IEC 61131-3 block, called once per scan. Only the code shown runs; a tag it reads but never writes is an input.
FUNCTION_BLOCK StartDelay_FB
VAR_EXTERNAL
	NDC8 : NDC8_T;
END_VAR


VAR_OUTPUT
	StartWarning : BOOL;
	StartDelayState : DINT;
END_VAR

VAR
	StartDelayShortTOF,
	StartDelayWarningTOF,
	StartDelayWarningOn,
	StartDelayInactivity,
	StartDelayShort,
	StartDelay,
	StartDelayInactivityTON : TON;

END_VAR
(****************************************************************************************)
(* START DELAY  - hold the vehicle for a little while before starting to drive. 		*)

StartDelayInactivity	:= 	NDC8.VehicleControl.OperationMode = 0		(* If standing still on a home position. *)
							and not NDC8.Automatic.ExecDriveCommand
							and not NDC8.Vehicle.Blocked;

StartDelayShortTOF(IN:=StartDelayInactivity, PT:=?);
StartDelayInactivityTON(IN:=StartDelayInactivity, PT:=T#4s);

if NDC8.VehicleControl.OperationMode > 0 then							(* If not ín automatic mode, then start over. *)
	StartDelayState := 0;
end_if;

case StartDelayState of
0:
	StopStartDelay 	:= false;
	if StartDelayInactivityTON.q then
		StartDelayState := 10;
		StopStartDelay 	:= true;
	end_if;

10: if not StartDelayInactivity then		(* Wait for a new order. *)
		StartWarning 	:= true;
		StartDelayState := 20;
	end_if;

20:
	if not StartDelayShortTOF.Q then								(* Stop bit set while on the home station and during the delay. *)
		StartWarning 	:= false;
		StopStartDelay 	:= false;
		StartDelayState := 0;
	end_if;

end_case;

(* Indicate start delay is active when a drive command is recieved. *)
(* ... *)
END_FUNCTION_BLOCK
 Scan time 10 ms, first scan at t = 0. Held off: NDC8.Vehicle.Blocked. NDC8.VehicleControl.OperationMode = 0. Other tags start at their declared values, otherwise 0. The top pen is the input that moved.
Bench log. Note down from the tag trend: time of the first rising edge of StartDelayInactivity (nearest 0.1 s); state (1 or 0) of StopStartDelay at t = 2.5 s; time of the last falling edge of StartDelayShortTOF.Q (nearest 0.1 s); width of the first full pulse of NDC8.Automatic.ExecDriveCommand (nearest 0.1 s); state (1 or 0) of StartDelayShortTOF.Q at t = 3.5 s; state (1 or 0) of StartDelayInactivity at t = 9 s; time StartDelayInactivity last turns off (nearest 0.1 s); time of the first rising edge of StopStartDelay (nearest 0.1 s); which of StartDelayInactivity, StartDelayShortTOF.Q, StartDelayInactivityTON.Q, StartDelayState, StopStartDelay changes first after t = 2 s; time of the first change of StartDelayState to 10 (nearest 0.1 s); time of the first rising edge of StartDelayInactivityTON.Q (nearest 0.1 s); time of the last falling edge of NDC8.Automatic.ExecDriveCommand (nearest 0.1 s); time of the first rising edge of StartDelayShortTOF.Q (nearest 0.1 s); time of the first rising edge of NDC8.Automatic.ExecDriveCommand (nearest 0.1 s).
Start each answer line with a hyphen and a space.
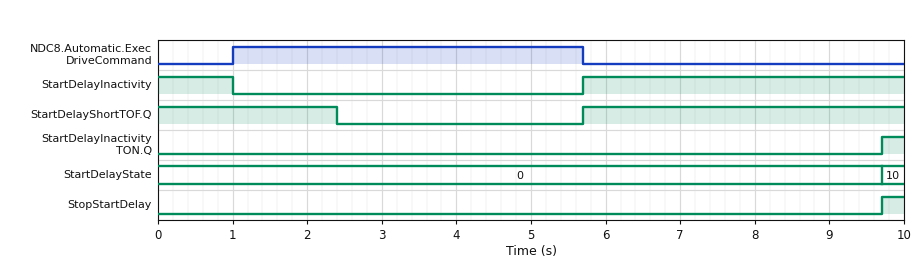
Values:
- 5.7 s
- 0
- 2.4 s
- 4.7 s
- 0
- 1
- 1.0 s
- 9.7 s
- StartDelayShortTOF.Q
- 9.7 s
- 9.7 s
- 5.7 s
- 5.7 s
- 1.0 s
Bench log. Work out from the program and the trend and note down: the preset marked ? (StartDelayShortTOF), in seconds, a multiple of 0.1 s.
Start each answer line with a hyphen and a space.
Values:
- 1.4 s
